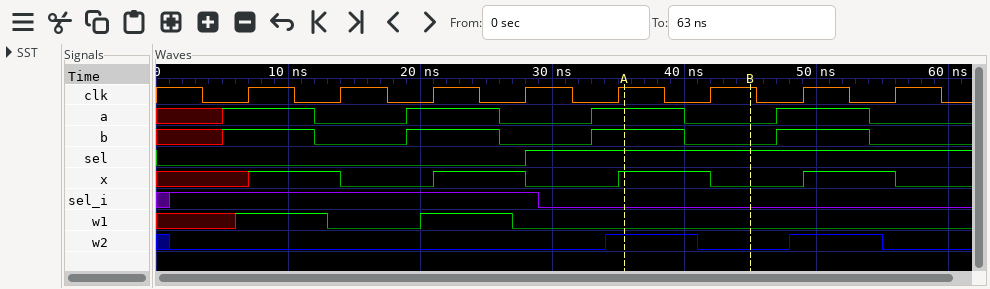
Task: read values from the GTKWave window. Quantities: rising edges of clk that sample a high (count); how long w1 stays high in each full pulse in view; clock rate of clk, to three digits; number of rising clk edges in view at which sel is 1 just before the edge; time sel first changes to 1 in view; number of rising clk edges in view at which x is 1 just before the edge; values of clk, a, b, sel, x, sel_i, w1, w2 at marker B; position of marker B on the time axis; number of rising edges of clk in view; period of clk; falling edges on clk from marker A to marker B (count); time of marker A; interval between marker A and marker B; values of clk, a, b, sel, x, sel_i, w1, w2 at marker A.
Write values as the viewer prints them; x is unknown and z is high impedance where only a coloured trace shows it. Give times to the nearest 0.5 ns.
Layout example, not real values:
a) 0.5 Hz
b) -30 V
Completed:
a) 4
b) 7 ns
c) 143 MHz
d) 4
e) 28 ns
f) 4
g) clk=1, a=0, b=0, sel=1, x=0, sel_i=0, w1=0, w2=0
h) 45 ns
i) 8
j) 7 ns
k) 1
l) 35.5 ns
m) 9.5 ns
n) clk=1, a=1, b=1, sel=1, x=1, sel_i=0, w1=0, w2=1
